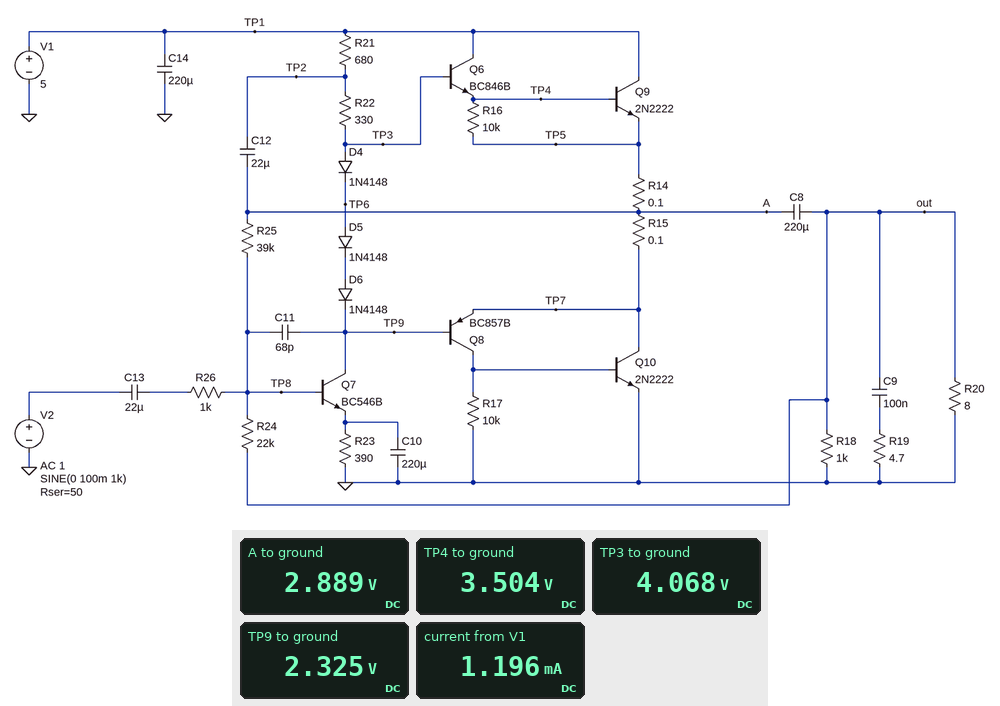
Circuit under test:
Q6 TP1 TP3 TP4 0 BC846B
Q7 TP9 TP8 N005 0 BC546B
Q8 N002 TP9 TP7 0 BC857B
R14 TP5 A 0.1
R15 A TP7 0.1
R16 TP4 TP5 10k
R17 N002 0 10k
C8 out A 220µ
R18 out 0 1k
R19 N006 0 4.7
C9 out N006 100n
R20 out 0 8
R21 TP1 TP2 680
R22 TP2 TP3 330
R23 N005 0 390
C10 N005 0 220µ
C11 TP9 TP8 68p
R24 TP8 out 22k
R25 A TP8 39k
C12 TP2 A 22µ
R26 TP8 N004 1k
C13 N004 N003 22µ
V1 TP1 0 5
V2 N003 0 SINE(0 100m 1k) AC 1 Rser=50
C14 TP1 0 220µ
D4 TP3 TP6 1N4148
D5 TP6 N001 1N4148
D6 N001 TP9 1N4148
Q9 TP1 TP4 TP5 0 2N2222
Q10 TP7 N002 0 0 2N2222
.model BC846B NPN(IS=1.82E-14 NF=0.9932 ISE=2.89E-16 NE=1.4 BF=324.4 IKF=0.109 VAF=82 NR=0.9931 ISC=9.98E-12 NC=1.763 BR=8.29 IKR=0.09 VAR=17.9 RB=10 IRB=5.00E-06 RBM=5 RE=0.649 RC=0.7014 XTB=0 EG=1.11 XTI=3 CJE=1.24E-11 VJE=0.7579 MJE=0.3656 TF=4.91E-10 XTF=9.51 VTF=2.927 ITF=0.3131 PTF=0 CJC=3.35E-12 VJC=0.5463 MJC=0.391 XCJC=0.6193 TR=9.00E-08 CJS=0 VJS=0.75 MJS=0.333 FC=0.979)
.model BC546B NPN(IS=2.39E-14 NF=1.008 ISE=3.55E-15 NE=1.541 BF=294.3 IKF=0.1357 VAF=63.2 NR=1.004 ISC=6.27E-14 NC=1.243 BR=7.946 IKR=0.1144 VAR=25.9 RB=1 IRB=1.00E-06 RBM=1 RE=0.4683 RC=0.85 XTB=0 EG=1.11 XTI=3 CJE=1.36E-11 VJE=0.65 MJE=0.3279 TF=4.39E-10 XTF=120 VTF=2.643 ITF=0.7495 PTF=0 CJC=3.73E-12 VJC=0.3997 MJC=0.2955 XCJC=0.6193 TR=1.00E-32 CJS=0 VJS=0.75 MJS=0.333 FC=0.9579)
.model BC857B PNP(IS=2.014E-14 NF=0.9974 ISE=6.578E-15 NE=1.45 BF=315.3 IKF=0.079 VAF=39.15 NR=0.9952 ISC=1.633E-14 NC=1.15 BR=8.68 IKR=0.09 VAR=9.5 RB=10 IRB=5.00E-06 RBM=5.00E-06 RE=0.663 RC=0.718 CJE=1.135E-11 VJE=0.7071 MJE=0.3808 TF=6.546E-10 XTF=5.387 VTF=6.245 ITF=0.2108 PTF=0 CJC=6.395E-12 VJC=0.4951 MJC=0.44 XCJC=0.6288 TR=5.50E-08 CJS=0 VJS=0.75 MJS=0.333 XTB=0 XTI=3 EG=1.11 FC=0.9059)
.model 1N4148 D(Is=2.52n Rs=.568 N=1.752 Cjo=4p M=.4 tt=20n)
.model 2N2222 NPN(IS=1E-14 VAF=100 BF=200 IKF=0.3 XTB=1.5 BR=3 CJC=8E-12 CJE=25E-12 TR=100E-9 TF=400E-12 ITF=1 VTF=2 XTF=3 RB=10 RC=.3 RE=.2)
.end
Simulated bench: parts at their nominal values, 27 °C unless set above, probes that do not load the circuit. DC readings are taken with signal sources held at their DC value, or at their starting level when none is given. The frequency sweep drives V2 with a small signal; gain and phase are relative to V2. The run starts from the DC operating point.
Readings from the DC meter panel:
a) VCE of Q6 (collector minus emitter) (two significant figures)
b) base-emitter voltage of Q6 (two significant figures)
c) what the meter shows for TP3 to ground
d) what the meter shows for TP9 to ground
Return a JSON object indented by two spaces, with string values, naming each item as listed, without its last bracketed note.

{
  "VCE of Q6 (collector minus emitter)": "1.5 V",
  "base-emitter voltage of Q6": "560 mV",
  "what the meter shows for TP3 to ground": "4.068 V",
  "what the meter shows for TP9 to ground": "2.325 V"
}
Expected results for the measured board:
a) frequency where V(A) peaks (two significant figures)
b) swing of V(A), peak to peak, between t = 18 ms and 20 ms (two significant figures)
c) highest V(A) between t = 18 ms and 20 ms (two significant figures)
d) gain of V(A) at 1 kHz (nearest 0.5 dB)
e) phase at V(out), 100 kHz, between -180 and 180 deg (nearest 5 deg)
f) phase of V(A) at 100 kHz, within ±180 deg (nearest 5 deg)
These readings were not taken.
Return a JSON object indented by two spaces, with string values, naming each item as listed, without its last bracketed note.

{
  "frequency where V(A) peaks": "25 Hz",
  "swing of V(A), peak to peak, between t = 18 ms and 20 ms": "2.1 V",
  "highest V(A) between t = 18 ms and 20 ms": "3.8 V",
  "gain of V(A) at 1 kHz": "16.5 dB",
  "phase at V(out), 100 kHz, between -180 and 180 deg": "125 deg",
  "phase of V(A) at 100 kHz, within ±180 deg": "125 deg"
}
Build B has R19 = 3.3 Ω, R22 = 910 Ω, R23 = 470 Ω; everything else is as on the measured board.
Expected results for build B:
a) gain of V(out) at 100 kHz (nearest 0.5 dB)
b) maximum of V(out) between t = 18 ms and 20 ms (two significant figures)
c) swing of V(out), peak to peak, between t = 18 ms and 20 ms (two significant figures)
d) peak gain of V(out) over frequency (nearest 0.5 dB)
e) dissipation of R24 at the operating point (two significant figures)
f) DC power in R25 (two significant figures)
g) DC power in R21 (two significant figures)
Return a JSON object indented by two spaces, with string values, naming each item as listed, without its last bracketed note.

{
  "gain of V(out) at 100 kHz": "3.0 dB",
  "maximum of V(out) between t = 18 ms and 20 ms": "1.2 V",
  "swing of V(out), peak to peak, between t = 18 ms and 20 ms": "2.4 V",
  "peak gain of V(out) over frequency": "8.0 dB",
  "dissipation of R24 at the operating point": "42 µW",
  "DC power in R25": "82 µW",
  "DC power in R21": "330 µW"
}
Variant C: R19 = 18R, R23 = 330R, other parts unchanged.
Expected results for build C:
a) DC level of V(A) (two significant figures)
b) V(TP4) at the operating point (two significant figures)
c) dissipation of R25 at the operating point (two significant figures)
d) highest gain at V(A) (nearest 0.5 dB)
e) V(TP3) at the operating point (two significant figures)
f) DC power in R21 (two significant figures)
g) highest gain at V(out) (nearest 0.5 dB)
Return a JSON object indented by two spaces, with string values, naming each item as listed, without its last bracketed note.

{
  "DC level of V(A)": "2.8 V",
  "V(TP4) at the operating point": "3.4 V",
  "dissipation of R25 at the operating point": "87 µW",
  "highest gain at V(A)": "26.5 dB",
  "V(TP3) at the operating point": "4.0 V",
  "DC power in R21": "670 µW",
  "highest gain at V(out)": "18.0 dB"
}
